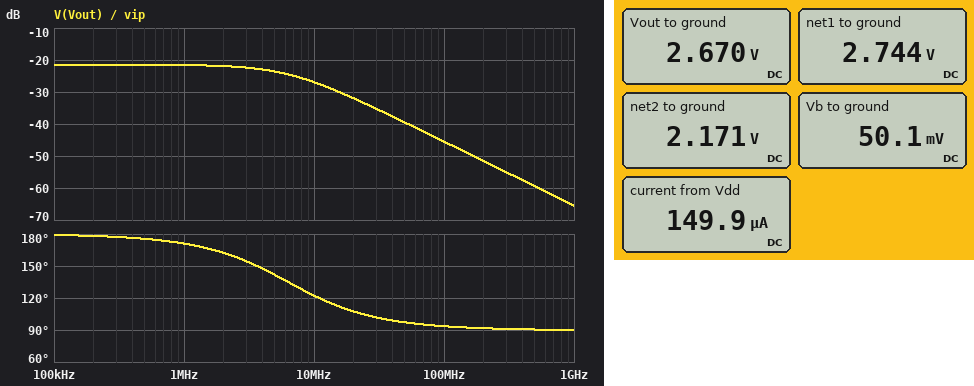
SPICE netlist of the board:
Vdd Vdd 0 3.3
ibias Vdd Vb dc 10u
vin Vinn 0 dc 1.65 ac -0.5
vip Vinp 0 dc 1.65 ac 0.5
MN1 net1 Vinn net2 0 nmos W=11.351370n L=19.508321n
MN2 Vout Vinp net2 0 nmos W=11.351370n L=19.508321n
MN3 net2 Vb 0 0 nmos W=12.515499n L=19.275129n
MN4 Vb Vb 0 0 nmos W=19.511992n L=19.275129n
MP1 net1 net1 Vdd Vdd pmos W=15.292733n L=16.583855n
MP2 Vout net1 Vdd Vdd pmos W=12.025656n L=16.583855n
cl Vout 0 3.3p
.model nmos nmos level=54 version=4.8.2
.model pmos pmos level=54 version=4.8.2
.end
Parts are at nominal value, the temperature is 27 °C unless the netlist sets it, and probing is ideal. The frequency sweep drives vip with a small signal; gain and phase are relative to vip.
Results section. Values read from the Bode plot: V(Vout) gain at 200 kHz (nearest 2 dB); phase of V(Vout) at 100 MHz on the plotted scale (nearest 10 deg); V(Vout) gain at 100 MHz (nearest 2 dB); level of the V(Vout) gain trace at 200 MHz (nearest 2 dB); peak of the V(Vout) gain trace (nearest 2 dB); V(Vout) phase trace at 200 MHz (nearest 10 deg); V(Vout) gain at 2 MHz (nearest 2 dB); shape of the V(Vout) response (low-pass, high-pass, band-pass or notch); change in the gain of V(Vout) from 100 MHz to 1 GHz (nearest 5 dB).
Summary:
-22 dB
90 deg
-46 dB
-52 dB
-22 dB
90 deg
-22 dB
low-pass
-20 dB
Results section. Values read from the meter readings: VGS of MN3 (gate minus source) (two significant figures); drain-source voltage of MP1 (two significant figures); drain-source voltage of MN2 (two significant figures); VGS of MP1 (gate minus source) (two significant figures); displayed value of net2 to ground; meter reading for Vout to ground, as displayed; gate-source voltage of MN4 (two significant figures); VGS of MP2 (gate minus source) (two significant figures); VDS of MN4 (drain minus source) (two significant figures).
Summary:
50 mV
-560 mV
500 mV
-560 mV
2.171 V
2.670 V
50 mV
-560 mV
50 mV
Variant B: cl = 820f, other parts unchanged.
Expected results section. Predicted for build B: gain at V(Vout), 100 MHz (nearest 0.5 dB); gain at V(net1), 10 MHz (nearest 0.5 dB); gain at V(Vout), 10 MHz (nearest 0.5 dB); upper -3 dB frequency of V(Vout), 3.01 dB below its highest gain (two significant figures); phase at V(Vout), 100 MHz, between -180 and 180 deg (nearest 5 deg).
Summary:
-33.5 dB
-27.5 dB
-22.0 dB
25 MHz
105 deg
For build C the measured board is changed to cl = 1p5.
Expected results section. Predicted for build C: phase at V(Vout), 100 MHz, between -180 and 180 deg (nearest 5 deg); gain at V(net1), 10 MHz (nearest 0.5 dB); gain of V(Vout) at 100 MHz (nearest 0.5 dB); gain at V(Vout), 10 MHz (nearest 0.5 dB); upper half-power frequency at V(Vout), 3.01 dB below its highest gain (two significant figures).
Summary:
100 deg
-27.5 dB
-38.5 dB
-23.5 dB
14 MHz
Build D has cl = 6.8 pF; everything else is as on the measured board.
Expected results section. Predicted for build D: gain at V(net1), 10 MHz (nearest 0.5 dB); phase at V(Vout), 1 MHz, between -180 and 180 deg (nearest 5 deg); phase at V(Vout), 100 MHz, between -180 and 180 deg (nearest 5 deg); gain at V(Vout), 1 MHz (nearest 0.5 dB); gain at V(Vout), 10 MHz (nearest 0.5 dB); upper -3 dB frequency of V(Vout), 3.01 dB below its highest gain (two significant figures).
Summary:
-26.5 dB
160 deg
90 deg
-22.0 dB
-32.0 dB
3.1 MHz
